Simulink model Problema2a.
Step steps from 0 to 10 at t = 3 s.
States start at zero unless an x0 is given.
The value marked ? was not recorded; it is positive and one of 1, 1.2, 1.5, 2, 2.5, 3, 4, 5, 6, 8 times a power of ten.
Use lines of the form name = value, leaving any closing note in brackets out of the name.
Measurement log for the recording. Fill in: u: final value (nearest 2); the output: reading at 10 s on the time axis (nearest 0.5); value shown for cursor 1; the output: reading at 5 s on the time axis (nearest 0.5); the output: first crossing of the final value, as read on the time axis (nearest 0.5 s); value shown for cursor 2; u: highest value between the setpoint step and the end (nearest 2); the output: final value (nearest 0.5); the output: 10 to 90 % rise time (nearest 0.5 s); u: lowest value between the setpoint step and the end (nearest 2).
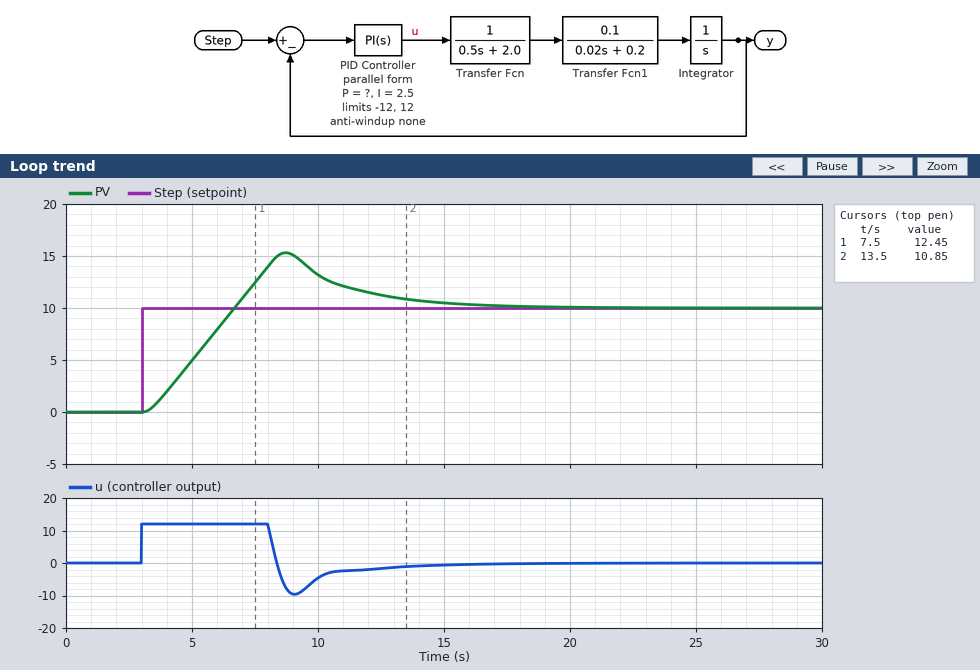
u: final value = 0
the output: reading at 10 s on the time axis = 13.0
value shown for cursor 1 = 12.45
the output: reading at 5 s on the time axis = 5.0
the output: first crossing of the final value, as read on the time axis = 6.5 s
value shown for cursor 2 = 10.85
u: highest value between the setpoint step and the end = 12
the output: final value = 10.0
the output: 10 to 90 % rise time = 2.5 s
u: lowest value between the setpoint step and the end = -10
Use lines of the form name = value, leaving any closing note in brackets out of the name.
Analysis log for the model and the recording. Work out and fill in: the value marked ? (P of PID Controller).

the value marked ? = 8
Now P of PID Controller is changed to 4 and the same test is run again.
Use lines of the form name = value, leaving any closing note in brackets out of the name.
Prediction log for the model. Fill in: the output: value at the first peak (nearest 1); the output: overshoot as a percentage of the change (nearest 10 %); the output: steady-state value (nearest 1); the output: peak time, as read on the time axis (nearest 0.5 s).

the output: value at the first peak = 17
the output: overshoot as a percentage of the change = 70 %
the output: steady-state value = 10
the output: peak time, as read on the time axis = 9.5 s
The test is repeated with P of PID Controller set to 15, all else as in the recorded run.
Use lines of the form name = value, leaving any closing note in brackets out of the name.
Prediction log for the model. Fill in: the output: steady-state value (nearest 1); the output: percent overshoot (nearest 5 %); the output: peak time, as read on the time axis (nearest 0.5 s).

the output: steady-state value = 10
the output: percent overshoot = 35 %
the output: peak time, as read on the time axis = 8.0 s
